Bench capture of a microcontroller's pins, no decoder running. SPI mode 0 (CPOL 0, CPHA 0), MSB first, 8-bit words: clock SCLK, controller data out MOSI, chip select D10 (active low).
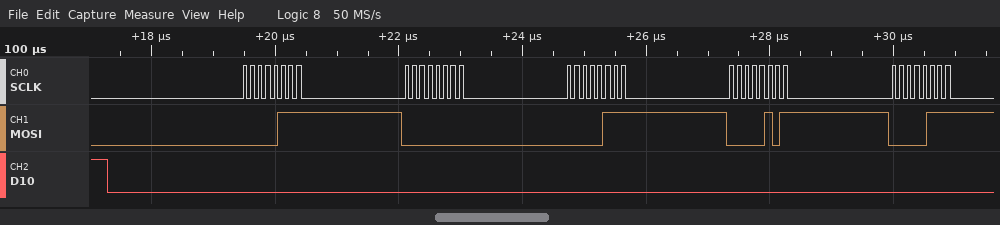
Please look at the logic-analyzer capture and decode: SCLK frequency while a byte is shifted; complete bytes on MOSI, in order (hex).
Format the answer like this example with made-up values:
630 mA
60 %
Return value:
8 MHz
07 00 07 05 07
